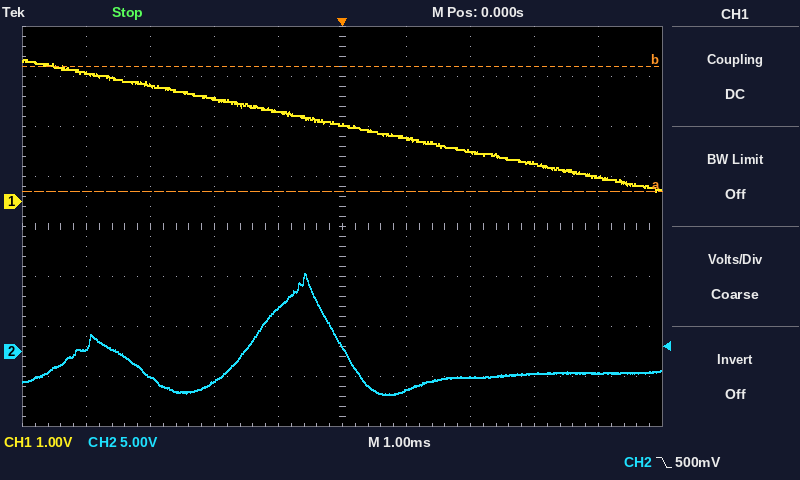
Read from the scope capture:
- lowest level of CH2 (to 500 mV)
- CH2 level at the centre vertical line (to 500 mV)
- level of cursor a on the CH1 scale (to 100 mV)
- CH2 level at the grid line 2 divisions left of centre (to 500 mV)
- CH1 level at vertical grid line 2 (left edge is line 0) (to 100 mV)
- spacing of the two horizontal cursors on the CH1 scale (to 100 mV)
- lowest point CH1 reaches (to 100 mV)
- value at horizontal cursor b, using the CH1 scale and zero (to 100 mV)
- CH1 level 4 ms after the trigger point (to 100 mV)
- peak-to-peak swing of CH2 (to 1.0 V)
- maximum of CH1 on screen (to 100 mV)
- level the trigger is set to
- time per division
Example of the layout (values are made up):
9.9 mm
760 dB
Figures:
-4.5 V
500 mV
200 mV
-3.0 V
2.3 V
2.5 V
200 mV
2.7 V
500 mV
12.0 V
2.8 V
500 mV
1 ms
